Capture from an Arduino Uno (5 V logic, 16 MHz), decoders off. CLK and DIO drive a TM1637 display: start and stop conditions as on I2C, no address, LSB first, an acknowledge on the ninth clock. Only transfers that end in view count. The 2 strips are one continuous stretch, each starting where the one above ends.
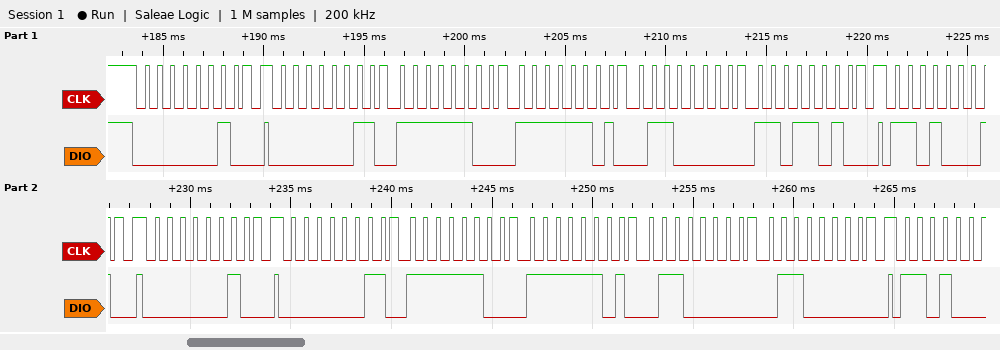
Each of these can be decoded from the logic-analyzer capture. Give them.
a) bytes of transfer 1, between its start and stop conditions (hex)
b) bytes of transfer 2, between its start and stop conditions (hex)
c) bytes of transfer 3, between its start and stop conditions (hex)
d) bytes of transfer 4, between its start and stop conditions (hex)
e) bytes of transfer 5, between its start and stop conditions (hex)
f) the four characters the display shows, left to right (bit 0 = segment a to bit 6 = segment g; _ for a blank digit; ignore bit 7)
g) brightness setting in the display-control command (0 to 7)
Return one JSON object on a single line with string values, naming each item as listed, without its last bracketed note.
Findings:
{"bytes of transfer 1, between its start and stop conditions": "40", "bytes of transfer 2, between its start and stop conditions": "C0 3F BF 06 5B", "bytes of transfer 3, between its start and stop conditions": "8B", "bytes of transfer 4, between its start and stop conditions": "40", "bytes of transfer 5, between its start and stop conditions": "C0 3F BF 06 06", "the four characters the display shows, left to right": "0011", "brightness setting in the display-control command": "3"}
